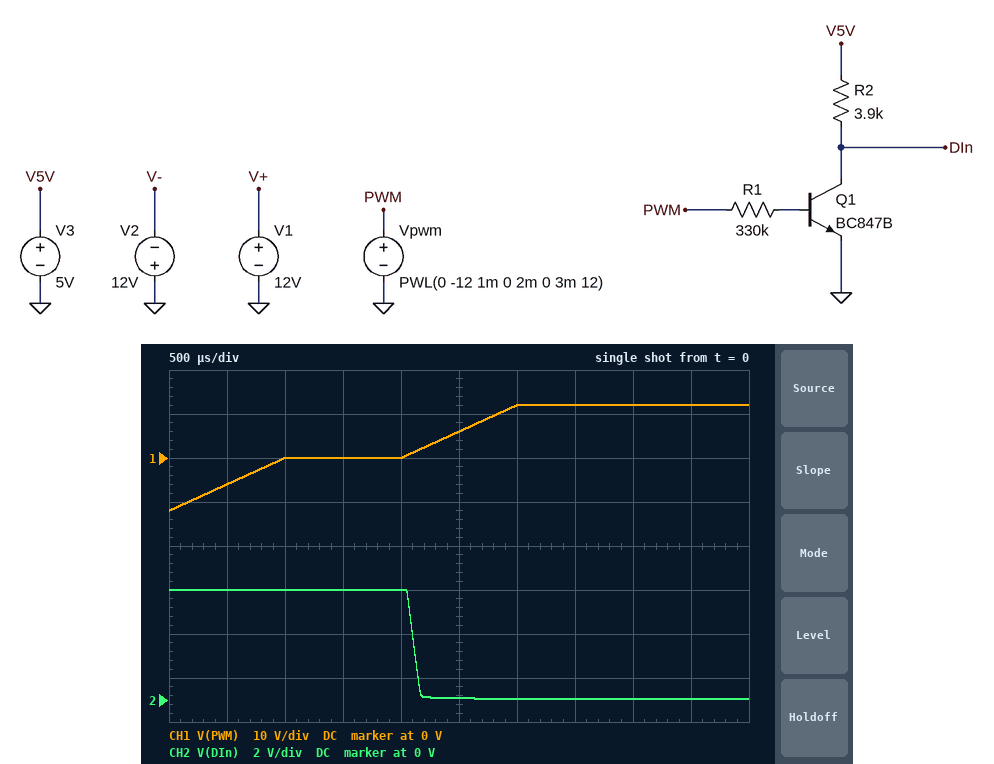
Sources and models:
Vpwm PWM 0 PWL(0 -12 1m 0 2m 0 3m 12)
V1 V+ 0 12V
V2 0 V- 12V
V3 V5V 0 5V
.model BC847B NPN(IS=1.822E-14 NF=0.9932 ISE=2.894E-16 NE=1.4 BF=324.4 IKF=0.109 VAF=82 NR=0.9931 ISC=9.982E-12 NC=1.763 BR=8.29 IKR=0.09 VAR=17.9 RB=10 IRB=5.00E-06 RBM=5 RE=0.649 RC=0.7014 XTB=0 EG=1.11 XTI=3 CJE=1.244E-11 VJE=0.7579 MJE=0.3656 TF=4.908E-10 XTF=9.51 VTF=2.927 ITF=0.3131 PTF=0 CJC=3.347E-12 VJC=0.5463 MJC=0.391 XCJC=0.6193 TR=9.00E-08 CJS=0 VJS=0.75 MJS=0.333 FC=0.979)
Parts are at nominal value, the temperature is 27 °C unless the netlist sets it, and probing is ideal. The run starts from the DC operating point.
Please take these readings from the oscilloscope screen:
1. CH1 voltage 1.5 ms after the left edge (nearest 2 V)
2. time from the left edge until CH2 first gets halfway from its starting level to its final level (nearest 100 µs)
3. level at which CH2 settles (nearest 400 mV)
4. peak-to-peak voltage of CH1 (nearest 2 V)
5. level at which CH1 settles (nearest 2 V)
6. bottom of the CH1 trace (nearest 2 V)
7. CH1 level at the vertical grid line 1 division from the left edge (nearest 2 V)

0 V
2.1 ms
0 V
24 V
12 V
-12 V
-6 V
